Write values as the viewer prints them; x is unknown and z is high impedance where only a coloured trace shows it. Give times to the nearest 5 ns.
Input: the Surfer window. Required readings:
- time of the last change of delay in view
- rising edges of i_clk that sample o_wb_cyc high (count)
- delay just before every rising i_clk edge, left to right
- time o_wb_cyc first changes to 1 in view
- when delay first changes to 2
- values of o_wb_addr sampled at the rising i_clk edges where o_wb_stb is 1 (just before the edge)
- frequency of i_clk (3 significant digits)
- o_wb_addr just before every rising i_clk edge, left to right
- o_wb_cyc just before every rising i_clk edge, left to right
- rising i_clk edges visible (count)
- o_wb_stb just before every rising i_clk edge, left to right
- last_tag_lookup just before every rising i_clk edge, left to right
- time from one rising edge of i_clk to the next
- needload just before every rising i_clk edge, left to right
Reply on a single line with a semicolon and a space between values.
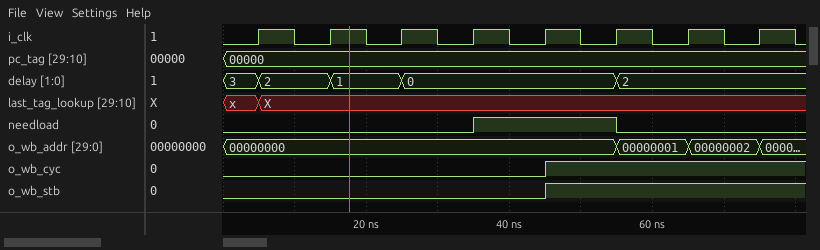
55 ns; 3; 3, 2, 1, 0, 0, 0, 2, 2; 45 ns; 5 ns; 00000000, 00000001, 00000002; 100 MHz; 00000000, 00000000, 00000000, 00000000, 00000000, 00000000, 00000001, 00000002; 0 0 0 0 0 1 1 1; 8; 0 0 0 0 0 1 1 1; x, X, X, X, X, X, X, X; 10 ns; 0 0 0 0 1 1 0 0
